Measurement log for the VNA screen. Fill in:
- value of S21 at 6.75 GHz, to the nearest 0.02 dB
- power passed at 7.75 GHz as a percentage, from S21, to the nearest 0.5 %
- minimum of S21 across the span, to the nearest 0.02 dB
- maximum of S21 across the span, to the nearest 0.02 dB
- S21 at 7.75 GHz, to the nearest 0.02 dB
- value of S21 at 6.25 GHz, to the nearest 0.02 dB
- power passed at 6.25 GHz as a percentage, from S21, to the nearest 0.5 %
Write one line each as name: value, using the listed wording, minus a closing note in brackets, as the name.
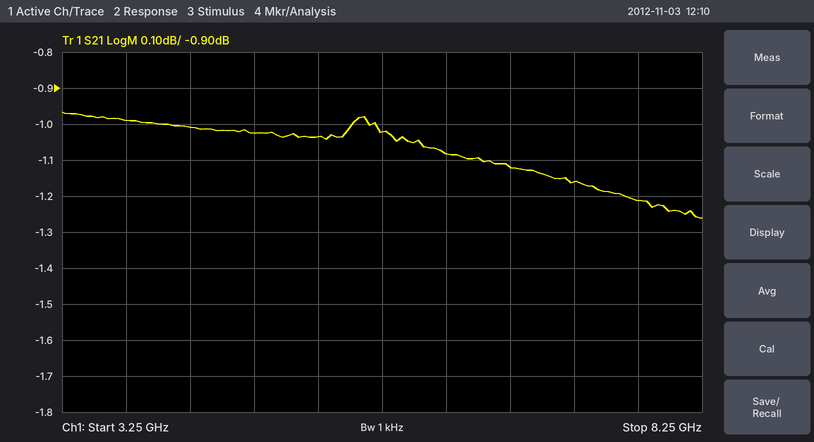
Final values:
value of S21 at 6.75 GHz, to the nearest 0.02 dB: -1.12 dB
power passed at 7.75 GHz as a percentage, from S21, to the nearest 0.5 %: 75.5 %
minimum of S21 across the span, to the nearest 0.02 dB: -1.26 dB
maximum of S21 across the span, to the nearest 0.02 dB: -0.96 dB
S21 at 7.75 GHz, to the nearest 0.02 dB: -1.22 dB
value of S21 at 6.25 GHz, to the nearest 0.02 dB: -1.08 dB
power passed at 6.25 GHz as a percentage, from S21, to the nearest 0.5 %: 78.0 %
